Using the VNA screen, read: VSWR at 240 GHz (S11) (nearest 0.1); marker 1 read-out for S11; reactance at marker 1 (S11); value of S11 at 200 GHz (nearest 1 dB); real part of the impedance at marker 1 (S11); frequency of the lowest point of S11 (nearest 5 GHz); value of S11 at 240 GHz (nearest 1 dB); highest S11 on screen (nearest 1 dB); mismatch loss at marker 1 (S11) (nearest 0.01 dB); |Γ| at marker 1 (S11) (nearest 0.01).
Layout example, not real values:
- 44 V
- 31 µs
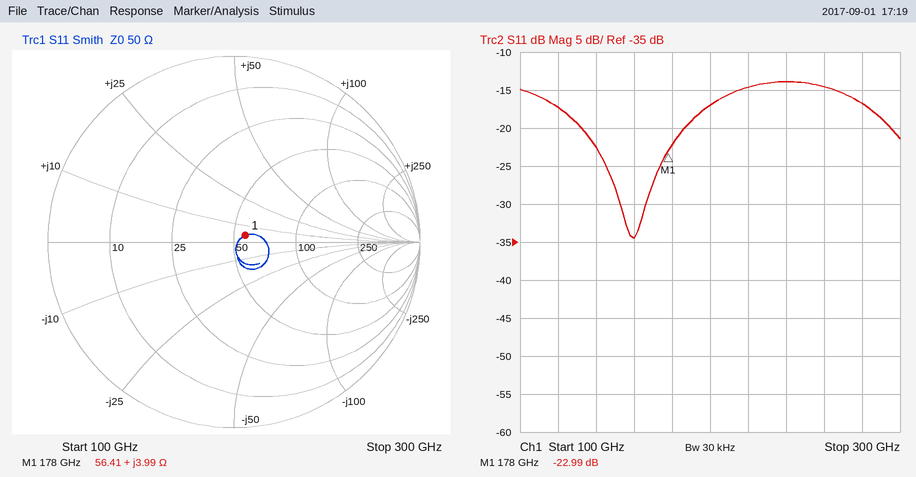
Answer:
- 1.5
- -22.99 dB
- +3.99 Ω
- -17 dB
- 56.41 Ω
- 160 GHz
- -14 dB
- -14 dB
- 0.02 dB
- 0.07
